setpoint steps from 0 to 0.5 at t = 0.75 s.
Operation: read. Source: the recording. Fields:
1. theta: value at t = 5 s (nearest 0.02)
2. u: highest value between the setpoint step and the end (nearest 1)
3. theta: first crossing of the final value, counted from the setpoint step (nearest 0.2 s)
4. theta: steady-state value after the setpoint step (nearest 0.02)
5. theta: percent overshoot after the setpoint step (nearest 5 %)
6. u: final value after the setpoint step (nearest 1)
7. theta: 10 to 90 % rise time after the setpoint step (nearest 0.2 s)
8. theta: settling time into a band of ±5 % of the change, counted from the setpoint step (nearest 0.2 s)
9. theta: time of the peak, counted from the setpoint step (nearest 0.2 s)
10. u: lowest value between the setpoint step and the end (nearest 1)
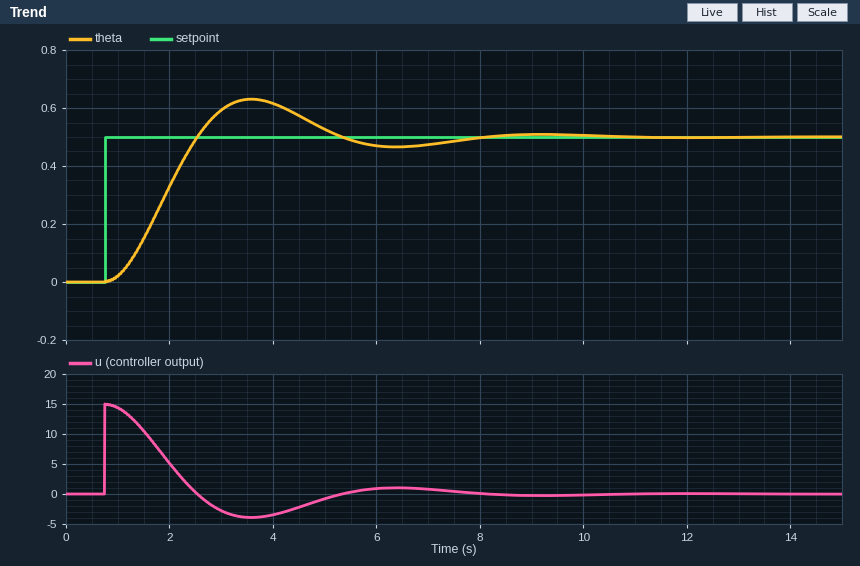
0.52
15
1.8 s
0.50
25 %
0
1.2 s
6.4 s
2.8 s
-4
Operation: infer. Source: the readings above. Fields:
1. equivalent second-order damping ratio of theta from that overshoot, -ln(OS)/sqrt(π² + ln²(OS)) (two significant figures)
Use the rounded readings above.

0.40
